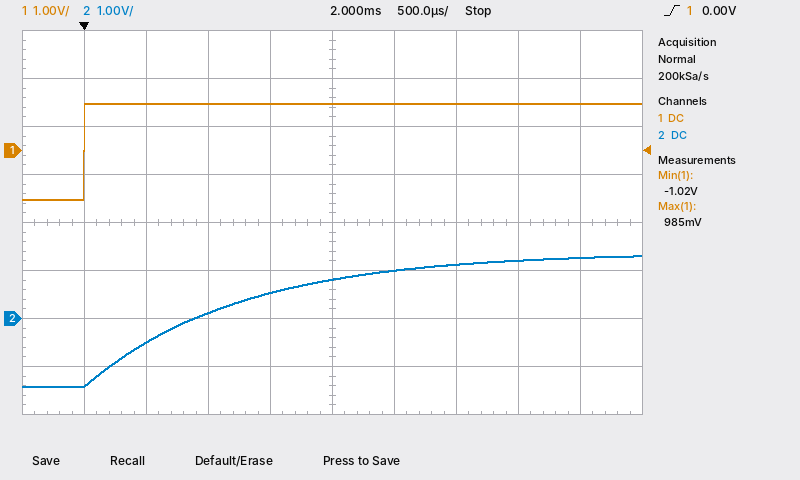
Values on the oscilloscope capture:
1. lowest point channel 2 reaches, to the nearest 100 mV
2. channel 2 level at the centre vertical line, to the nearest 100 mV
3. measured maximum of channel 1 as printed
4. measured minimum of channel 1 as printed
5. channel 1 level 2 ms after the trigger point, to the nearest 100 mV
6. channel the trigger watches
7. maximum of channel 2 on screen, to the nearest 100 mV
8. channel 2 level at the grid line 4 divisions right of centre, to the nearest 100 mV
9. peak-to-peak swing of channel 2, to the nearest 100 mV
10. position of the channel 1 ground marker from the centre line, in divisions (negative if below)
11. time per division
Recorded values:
-1.4 V
800 mV
985 mV
-1.02 V
1.0 V
channel 1
1.3 V
1.3 V
2.7 V
+1.5 div
500 µs
